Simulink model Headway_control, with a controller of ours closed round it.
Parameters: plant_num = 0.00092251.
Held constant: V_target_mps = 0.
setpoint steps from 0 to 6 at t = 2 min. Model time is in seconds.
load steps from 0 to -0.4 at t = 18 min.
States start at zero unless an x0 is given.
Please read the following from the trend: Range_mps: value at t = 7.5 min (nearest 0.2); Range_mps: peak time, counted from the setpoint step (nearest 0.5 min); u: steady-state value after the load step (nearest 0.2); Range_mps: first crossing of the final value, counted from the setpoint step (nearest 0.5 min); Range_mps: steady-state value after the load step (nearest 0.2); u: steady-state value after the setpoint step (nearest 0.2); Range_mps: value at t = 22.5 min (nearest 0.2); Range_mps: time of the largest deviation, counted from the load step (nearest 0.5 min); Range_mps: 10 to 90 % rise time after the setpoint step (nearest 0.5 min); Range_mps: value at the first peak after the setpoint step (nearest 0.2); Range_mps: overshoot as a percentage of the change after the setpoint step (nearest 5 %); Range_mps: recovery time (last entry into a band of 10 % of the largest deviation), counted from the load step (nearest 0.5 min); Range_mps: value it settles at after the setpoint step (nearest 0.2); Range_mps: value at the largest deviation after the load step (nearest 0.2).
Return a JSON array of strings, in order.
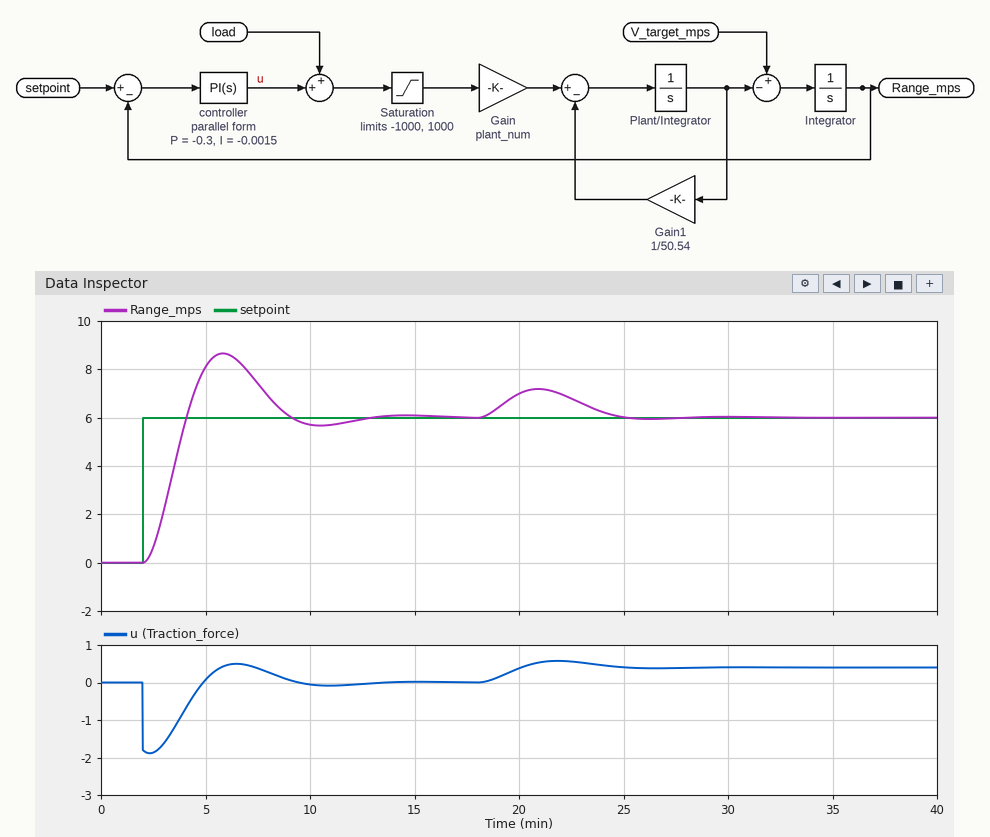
["7.4", "4.0 min", "0.4", "2.0 min", "6.0", "0.0", "6.8", "3.0 min", "1.5 min", "8.6", "45 %", "6.5 min", "6.0", "7.2"]
